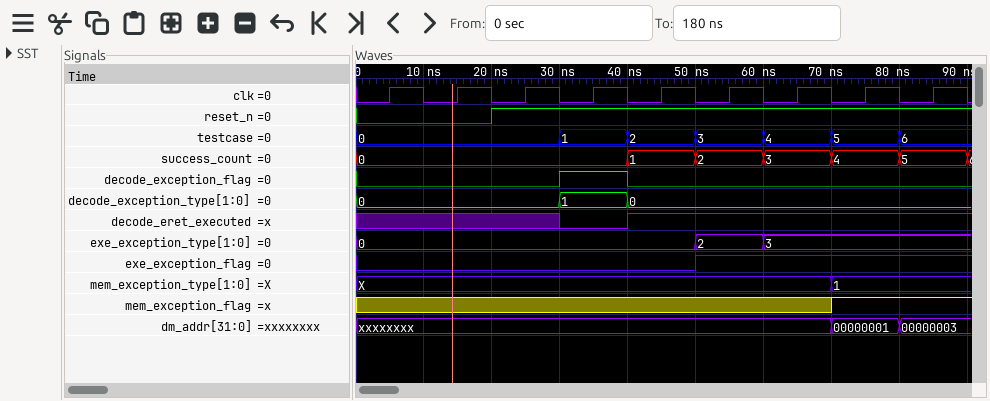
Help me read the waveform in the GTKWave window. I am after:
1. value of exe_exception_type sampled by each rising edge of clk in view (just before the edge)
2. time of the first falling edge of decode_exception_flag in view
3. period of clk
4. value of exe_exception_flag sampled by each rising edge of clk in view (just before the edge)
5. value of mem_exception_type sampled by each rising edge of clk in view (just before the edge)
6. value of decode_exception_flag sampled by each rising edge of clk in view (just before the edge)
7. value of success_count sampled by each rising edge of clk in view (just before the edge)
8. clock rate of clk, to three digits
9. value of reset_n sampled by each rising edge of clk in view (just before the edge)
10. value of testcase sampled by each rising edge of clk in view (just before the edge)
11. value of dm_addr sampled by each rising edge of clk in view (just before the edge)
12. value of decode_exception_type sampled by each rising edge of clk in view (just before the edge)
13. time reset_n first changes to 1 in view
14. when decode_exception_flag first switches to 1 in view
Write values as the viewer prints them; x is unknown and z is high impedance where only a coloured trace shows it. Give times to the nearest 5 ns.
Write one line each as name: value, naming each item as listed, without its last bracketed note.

value of exe_exception_type sampled by each rising edge of clk in view: 0, 0, 0, 0, 0, 2, 3, 3, 3
time of the first falling edge of decode_exception_flag in view: 40 ns
period of clk: 10 ns
value of exe_exception_flag sampled by each rising edge of clk in view: 0 0 0 0 0 1 1 1 1
value of mem_exception_type sampled by each rising edge of clk in view: X, X, X, X, X, X, X, 1, 1
value of decode_exception_flag sampled by each rising edge of clk in view: 0 0 0 1 0 0 0 0 0
value of success_count sampled by each rising edge of clk in view: 0, 0, 0, 0, 1, 2, 3, 4, 5
clock rate of clk, to three digits: 100 MHz
value of reset_n sampled by each rising edge of clk in view: 0 0 1 1 1 1 1 1 1
value of testcase sampled by each rising edge of clk in view: 0, 0, 0, 1, 2, 3, 4, 5, 6
value of dm_addr sampled by each rising edge of clk in view: xxxxxxxx, xxxxxxxx, xxxxxxxx, xxxxxxxx, xxxxxxxx, xxxxxxxx, xxxxxxxx, 00000001, 00000003
value of decode_exception_type sampled by each rising edge of clk in view: 0, 0, 0, 1, 0, 0, 0, 0, 0
time reset_n first changes to 1 in view: 20 ns
when decode_exception_flag first switches to 1 in view: 30 ns
